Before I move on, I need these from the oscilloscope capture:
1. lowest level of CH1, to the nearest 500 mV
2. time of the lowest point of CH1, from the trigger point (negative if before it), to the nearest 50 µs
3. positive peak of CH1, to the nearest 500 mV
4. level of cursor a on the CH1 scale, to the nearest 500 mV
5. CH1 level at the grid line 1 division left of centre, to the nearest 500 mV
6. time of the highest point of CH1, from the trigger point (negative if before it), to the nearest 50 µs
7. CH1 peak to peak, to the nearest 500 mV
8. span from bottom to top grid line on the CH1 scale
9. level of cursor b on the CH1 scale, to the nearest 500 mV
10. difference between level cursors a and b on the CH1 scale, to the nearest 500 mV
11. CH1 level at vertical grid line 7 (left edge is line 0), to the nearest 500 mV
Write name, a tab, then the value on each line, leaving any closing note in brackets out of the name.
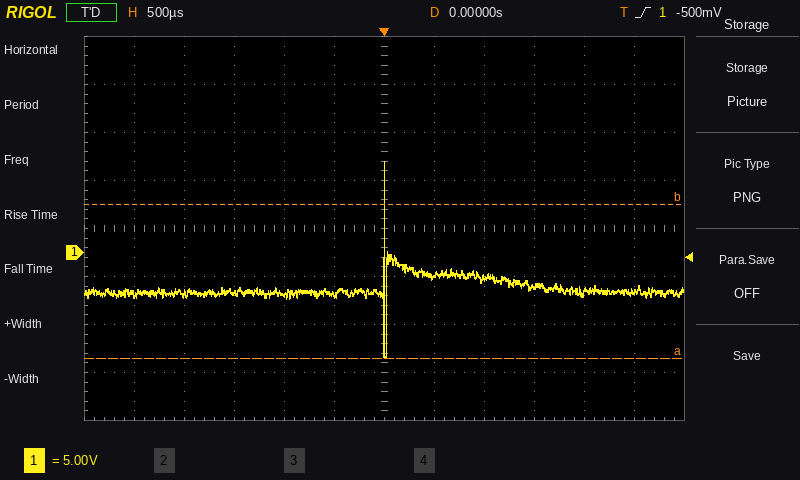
lowest level of CH1, to the nearest 500 mV	-11.0 V
time of the lowest point of CH1, from the trigger point (negative if before it), to the nearest 50 µs	0 µs
positive peak of CH1, to the nearest 500 mV	9.5 V
level of cursor a on the CH1 scale, to the nearest 500 mV	-11.0 V
CH1 level at the grid line 1 division left of centre, to the nearest 500 mV	-4.5 V
time of the highest point of CH1, from the trigger point (negative if before it), to the nearest 50 µs	0 µs
CH1 peak to peak, to the nearest 500 mV	20.5 V
span from bottom to top grid line on the CH1 scale	40 V
level of cursor b on the CH1 scale, to the nearest 500 mV	5.0 V
difference between level cursors a and b on the CH1 scale, to the nearest 500 mV	16.0 V
CH1 level at vertical grid line 7 (left edge is line 0), to the nearest 500 mV	-2.5 V
